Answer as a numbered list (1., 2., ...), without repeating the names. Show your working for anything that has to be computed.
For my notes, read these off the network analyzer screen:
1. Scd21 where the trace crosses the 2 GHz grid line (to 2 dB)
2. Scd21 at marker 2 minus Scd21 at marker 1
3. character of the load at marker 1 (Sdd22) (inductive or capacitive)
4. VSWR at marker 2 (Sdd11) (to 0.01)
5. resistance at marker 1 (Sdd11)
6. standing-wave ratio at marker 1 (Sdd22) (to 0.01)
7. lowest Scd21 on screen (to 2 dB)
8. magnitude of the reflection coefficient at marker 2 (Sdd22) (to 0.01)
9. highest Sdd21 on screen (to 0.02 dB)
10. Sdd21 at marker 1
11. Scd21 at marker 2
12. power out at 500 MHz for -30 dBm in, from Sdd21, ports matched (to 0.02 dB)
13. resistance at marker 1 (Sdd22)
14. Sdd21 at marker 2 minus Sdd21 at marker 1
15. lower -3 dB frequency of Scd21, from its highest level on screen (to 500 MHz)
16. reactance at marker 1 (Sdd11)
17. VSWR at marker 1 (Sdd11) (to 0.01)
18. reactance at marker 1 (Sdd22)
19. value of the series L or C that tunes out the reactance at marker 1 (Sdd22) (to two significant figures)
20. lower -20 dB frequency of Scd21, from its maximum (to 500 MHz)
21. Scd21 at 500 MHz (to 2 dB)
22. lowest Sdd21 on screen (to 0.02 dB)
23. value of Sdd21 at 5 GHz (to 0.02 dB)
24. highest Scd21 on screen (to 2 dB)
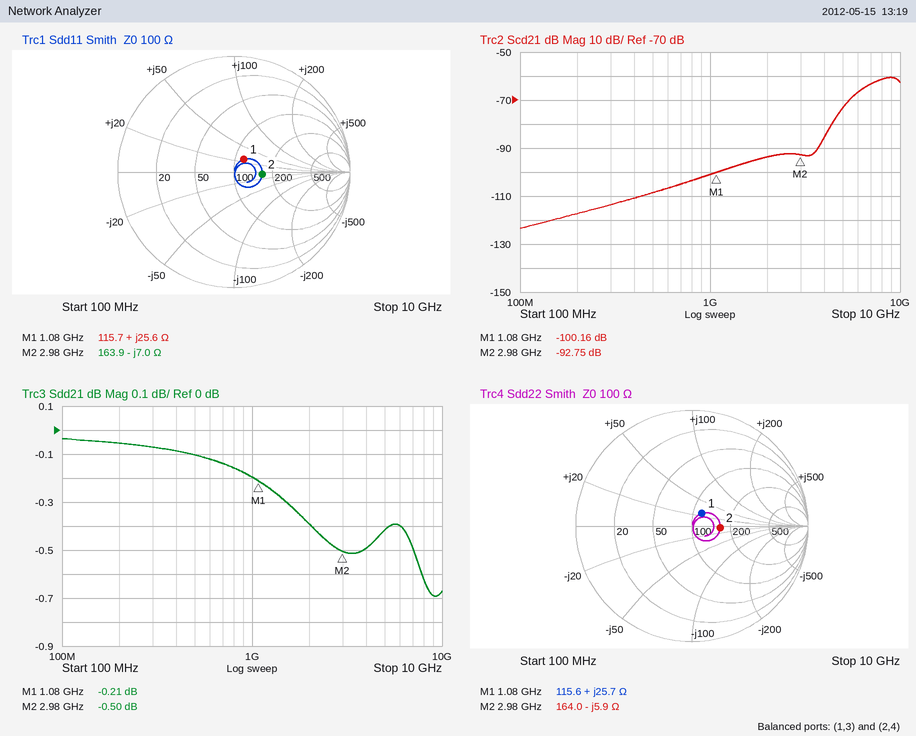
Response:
1. -94 dB
2. -92.75 − (-100.16) = 7.41 dB
3. inductive
4. 1.64
5. 115.7 Ω
6. 1.32
7. -124 dB
8. 0.24
9. -0.04 dB
10. -0.21 dB
11. -92.75 dB
12. -30 dBm + (-0.10 dB) = -30.10 dBm
13. 115.6 Ω
14. -0.5 − (-0.21) = -0.29 dB
15. 7.0 GHz
16. +25.6 Ω
17. 1.32
18. +25.7 Ω
19. C = 1/(2π × 1.08 GHz × 25.7 Ω) ≈ 5.7 pF
20. 4.5 GHz
21. -108 dB
22. -0.70 dB
23. -0.42 dB
24. -60 dB
